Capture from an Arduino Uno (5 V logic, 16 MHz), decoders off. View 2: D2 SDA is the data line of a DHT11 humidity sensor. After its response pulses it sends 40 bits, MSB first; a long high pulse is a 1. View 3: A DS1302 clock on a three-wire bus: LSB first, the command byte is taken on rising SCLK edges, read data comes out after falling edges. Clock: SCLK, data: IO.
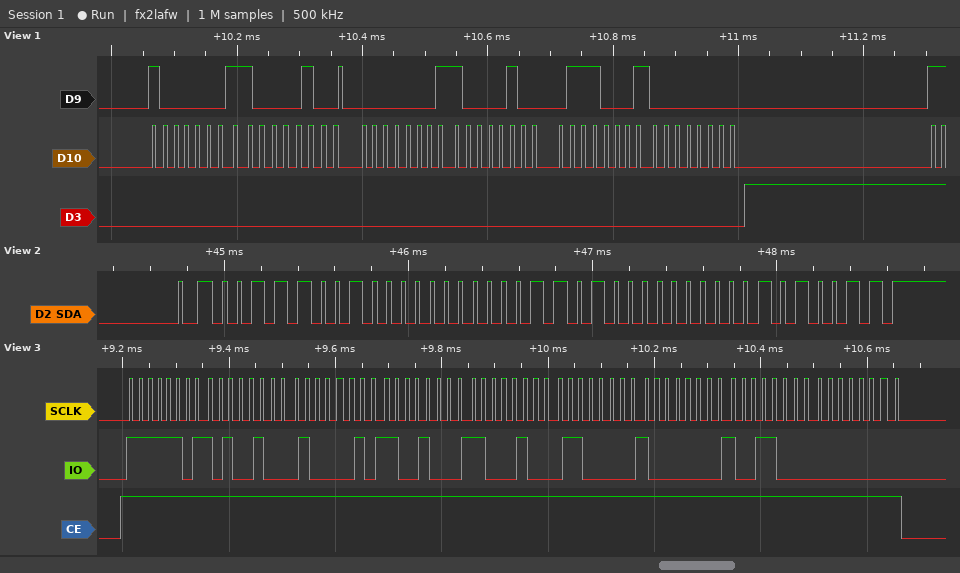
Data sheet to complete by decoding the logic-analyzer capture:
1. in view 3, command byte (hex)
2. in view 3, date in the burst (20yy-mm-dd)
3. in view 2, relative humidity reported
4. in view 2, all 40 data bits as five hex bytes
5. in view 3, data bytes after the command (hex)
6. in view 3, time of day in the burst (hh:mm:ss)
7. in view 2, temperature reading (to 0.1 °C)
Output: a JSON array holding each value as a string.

["0xBF", "2019-06-23", "57 %", "39 00 1A 00 53", "25 42 13 23 06 01 19 00", "13:42:25", "26.0 °C"]
